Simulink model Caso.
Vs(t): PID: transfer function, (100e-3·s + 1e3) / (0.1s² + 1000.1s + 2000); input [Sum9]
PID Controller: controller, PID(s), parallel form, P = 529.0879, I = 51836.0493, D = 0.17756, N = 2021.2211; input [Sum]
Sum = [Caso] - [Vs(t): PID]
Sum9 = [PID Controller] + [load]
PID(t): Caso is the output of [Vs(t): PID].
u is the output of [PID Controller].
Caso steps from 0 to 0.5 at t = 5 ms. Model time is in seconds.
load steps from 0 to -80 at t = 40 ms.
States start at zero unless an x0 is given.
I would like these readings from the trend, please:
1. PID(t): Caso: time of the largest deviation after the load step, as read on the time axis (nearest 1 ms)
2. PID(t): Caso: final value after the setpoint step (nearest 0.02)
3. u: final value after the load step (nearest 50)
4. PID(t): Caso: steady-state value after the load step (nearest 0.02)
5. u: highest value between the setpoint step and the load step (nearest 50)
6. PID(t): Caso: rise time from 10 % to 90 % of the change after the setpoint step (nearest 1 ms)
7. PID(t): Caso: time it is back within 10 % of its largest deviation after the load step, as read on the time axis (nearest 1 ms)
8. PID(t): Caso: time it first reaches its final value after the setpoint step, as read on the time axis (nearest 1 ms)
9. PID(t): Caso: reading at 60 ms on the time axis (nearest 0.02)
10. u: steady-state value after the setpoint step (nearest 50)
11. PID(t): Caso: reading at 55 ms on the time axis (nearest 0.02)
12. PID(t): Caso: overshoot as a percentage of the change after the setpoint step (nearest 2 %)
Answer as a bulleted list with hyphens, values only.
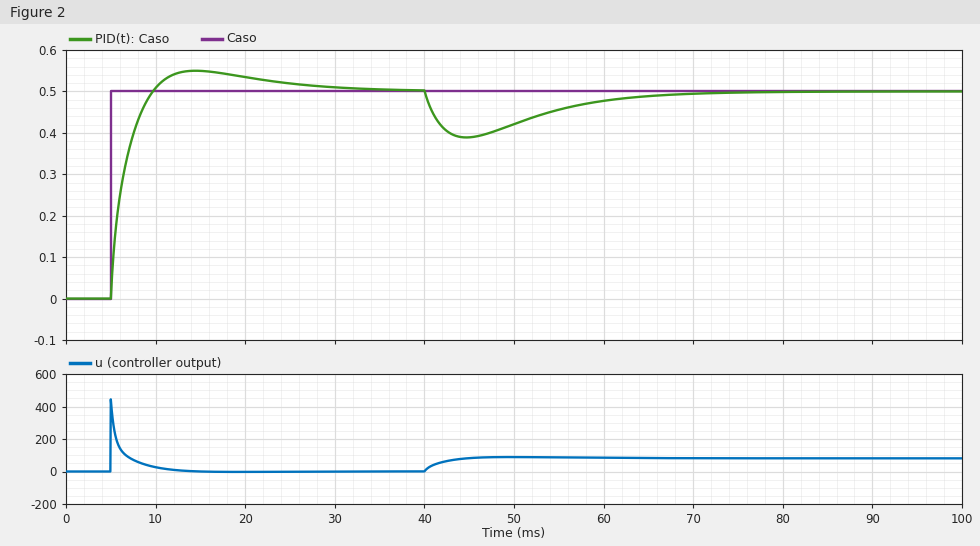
- 45 ms
- 0.50
- 100
- 0.50
- 450
- 3 ms
- 65 ms
- 10 ms
- 0.48
- 0
- 0.46
- 10 %
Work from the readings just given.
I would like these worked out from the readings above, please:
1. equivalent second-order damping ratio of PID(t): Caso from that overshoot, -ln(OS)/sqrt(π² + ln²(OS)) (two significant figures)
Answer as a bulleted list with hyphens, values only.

- 0.59
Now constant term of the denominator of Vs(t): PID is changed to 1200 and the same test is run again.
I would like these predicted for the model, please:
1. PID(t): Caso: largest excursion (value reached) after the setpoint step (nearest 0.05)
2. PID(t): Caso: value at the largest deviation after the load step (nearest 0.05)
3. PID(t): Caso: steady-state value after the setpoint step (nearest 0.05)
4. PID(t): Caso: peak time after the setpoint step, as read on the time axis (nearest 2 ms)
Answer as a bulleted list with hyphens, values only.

- 0.55
- 0.40
- 0.50
- 14 ms
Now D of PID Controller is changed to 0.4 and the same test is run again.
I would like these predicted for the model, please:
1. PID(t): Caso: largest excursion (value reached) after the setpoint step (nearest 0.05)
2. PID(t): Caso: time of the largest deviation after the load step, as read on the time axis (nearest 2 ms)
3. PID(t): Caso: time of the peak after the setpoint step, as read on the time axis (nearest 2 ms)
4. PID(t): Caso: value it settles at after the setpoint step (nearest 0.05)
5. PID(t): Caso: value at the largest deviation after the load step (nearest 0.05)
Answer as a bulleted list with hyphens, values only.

- 0.55
- 46 ms
- 16 ms
- 0.50
- 0.40
